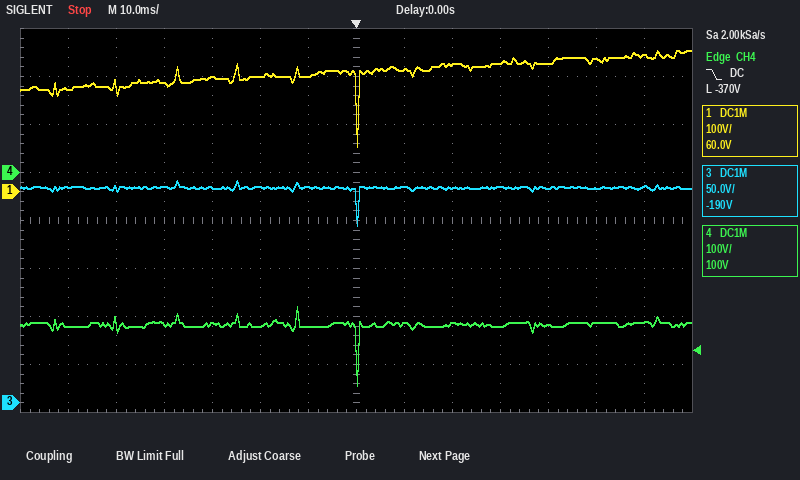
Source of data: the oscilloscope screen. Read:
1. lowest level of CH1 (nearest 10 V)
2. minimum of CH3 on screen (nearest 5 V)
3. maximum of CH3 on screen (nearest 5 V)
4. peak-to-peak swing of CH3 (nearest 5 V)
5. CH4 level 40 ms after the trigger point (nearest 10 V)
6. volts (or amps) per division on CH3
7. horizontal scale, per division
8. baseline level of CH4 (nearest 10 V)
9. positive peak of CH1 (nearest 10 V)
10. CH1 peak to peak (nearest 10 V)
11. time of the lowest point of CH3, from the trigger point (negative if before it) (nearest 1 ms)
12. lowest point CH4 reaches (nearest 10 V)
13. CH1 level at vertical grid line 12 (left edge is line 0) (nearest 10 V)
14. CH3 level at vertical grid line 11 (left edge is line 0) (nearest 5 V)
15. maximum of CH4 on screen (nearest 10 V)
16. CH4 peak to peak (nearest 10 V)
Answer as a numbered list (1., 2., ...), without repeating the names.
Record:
1. 90 V
2. 185 V
3. 230 V
4. 45 V
5. -320 V
6. 50 V
7. 10 ms
8. -320 V
9. 290 V
10. 200 V
11. 0 ms
12. -440 V
13. 280 V
14. 225 V
15. -280 V
16. 160 V
